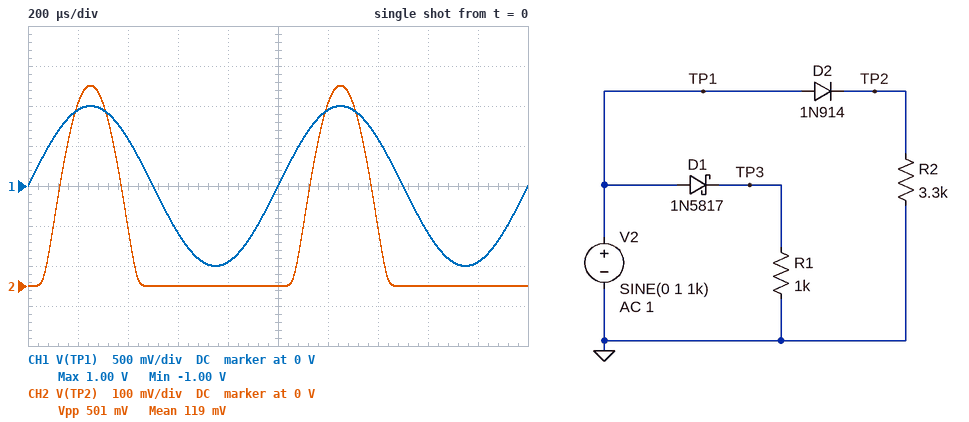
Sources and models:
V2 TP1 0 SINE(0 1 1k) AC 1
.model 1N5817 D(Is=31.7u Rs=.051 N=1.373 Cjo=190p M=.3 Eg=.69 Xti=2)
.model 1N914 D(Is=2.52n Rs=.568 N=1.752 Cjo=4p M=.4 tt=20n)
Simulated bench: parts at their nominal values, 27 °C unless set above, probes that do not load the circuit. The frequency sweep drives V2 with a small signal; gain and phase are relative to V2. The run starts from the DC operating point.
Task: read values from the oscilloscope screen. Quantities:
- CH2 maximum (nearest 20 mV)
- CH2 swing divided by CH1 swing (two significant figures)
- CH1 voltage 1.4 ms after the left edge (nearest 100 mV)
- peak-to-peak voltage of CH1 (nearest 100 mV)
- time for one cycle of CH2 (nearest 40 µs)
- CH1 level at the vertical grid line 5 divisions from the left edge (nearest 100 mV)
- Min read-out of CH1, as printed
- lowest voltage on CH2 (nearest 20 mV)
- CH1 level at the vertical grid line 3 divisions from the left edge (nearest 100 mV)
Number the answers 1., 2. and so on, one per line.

1. 500 mV
2. 0.25
3. 600 mV
4. 2.0 V
5. 1.00 ms
6. 0 V
7. -1.00 V
8. 0 V
9. -600 mV
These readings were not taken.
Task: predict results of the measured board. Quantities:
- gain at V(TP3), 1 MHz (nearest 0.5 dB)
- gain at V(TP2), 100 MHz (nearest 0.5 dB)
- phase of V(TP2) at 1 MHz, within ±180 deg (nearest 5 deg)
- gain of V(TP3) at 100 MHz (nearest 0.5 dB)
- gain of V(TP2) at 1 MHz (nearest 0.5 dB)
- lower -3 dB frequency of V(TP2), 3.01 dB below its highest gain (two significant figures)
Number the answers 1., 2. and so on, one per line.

1. -3.5 dB
2. 0 dB
3. 85 deg
4. 0 dB
5. -21.5 dB
6. 12 MHz
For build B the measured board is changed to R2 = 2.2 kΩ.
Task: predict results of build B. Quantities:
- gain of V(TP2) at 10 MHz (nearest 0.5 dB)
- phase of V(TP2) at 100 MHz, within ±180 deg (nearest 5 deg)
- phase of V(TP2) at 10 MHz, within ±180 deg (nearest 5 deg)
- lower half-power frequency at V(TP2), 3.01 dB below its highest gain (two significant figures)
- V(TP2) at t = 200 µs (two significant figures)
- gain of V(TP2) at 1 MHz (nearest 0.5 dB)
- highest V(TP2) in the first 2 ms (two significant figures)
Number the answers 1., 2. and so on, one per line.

1. -6.5 dB
2. 10 deg
3. 60 deg
4. 18 MHz
5. 440 mV
6. -25.0 dB
7. 480 mV
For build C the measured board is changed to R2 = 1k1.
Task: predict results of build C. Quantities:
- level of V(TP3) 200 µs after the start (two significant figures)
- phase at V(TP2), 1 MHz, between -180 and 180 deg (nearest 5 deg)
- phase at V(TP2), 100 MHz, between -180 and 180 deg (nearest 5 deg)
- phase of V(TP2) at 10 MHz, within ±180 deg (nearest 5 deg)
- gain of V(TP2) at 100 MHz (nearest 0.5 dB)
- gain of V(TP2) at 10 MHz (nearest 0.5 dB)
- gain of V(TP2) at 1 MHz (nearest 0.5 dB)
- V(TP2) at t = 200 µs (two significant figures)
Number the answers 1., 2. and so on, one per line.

1. 830 mV
2. 90 deg
3. 20 deg
4. 75 deg
5. -0.5 dB
6. -11.5 dB
7. -31.0 dB
8. 410 mV
